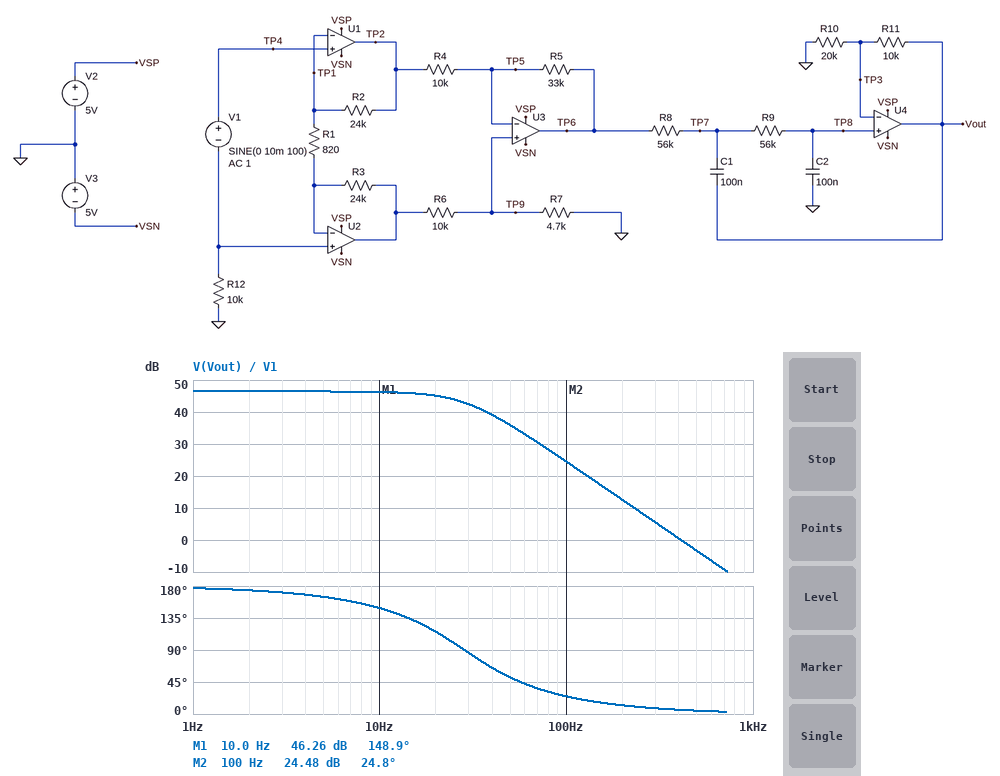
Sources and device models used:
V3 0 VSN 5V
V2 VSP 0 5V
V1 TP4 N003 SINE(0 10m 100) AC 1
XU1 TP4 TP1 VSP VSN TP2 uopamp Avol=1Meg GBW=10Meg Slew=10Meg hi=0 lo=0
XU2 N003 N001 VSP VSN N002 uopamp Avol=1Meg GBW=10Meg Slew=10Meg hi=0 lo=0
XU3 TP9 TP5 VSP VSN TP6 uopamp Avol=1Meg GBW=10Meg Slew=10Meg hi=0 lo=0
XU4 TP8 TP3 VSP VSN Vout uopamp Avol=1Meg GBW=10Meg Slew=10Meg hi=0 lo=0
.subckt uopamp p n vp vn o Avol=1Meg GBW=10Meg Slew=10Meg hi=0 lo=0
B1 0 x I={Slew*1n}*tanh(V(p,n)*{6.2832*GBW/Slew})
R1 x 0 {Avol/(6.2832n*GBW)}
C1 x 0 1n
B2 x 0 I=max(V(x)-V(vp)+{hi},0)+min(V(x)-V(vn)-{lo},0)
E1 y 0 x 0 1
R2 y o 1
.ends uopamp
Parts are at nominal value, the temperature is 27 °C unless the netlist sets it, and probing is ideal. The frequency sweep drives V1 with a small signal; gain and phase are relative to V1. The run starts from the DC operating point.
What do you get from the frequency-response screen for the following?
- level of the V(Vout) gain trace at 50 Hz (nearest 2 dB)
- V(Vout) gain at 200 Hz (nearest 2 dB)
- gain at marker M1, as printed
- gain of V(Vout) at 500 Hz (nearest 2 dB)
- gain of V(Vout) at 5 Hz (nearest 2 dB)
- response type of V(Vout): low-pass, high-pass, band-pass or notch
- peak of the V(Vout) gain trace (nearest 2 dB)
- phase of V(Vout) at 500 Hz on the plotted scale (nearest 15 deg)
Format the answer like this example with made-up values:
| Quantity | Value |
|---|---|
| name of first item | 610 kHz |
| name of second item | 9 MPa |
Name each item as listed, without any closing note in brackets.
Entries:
| Quantity | Value |
|---|---|
| level of the V(Vout) gain trace at 50 Hz | 36 dB |
| V(Vout) gain at 200 Hz | 12 dB |
| gain at marker M1, as printed | 46.26 dB |
| gain of V(Vout) at 500 Hz | -4 dB |
| gain of V(Vout) at 5 Hz | 46 dB |
| response type of V(Vout): low-pass, high-pass, band-pass or notch | low-pass |
| peak of the V(Vout) gain trace | 46 dB |
| phase of V(Vout) at 500 Hz on the plotted scale | 0 deg |
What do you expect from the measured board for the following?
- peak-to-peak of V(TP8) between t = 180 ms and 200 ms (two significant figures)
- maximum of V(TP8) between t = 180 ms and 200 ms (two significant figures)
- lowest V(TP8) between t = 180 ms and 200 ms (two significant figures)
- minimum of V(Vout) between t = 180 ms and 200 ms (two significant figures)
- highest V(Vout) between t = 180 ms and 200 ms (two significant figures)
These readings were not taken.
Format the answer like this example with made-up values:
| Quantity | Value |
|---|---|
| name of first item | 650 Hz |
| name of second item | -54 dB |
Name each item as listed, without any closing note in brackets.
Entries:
| Quantity | Value |
|---|---|
| peak-to-peak of V(TP8) between t = 180 ms and 200 ms | 220 mV |
| maximum of V(TP8) between t = 180 ms and 200 ms | 110 mV |
| lowest V(TP8) between t = 180 ms and 200 ms | -110 mV |
| minimum of V(Vout) between t = 180 ms and 200 ms | -170 mV |
| highest V(Vout) between t = 180 ms and 200 ms | 170 mV |
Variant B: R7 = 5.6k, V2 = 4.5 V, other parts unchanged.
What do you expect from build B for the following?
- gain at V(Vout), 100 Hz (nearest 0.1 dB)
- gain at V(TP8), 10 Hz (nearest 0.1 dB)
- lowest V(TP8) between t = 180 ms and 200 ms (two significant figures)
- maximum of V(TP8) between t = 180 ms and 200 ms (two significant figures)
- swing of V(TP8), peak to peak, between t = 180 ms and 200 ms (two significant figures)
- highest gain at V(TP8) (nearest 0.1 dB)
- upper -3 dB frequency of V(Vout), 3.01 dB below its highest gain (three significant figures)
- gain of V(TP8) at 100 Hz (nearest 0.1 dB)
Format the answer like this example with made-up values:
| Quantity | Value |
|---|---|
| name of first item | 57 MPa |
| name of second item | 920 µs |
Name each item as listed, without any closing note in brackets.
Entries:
| Quantity | Value |
|---|---|
| gain at V(Vout), 100 Hz | 24.8 dB |
| gain at V(TP8), 10 Hz | 43.0 dB |
| lowest V(TP8) between t = 180 ms and 200 ms | -120 mV |
| maximum of V(TP8) between t = 180 ms and 200 ms | 120 mV |
| swing of V(TP8), peak to peak, between t = 180 ms and 200 ms | 230 mV |
| highest gain at V(TP8) | 43.2 dB |
| upper -3 dB frequency of V(Vout), 3.01 dB below its highest gain | 26.7 Hz |
| gain of V(TP8) at 100 Hz | 21.3 dB |
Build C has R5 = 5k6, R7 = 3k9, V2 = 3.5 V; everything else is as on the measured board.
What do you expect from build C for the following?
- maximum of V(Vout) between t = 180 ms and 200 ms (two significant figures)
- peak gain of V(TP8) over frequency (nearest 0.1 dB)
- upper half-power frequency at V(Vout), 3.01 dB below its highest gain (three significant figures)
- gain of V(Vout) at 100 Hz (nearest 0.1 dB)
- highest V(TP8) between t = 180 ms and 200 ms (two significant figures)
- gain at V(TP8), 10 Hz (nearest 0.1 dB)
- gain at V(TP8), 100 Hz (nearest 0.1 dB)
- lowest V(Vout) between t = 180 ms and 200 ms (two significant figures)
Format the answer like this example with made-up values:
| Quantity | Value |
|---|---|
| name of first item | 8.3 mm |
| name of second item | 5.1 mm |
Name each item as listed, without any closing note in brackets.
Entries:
| Quantity | Value |
|---|---|
| maximum of V(Vout) between t = 180 ms and 200 ms | 36 mV |
| peak gain of V(TP8) over frequency | 29.5 dB |
| upper half-power frequency at V(Vout), 3.01 dB below its highest gain | 26.7 Hz |
| gain of V(Vout) at 100 Hz | 11.0 dB |
| highest V(TP8) between t = 180 ms and 200 ms | 24 mV |
| gain at V(TP8), 10 Hz | 29.3 dB |
| gain at V(TP8), 100 Hz | 7.5 dB |
| lowest V(Vout) between t = 180 ms and 200 ms | -36 mV |
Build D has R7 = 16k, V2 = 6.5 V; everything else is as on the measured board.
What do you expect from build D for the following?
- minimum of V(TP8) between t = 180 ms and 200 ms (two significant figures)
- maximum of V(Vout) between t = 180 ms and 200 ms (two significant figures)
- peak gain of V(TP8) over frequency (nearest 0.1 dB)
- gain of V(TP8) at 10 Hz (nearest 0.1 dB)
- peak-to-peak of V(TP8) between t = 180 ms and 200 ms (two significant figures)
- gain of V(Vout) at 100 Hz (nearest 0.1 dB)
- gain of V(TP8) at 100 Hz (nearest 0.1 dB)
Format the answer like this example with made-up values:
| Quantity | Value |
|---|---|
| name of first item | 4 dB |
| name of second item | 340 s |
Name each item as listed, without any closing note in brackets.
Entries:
| Quantity | Value |
|---|---|
| minimum of V(TP8) between t = 180 ms and 200 ms | -140 mV |
| maximum of V(Vout) between t = 180 ms and 200 ms | 210 mV |
| peak gain of V(TP8) over frequency | 45.0 dB |
| gain of V(TP8) at 10 Hz | 44.8 dB |
| peak-to-peak of V(TP8) between t = 180 ms and 200 ms | 280 mV |
| gain of V(Vout) at 100 Hz | 26.5 dB |
| gain of V(TP8) at 100 Hz | 23.0 dB |
